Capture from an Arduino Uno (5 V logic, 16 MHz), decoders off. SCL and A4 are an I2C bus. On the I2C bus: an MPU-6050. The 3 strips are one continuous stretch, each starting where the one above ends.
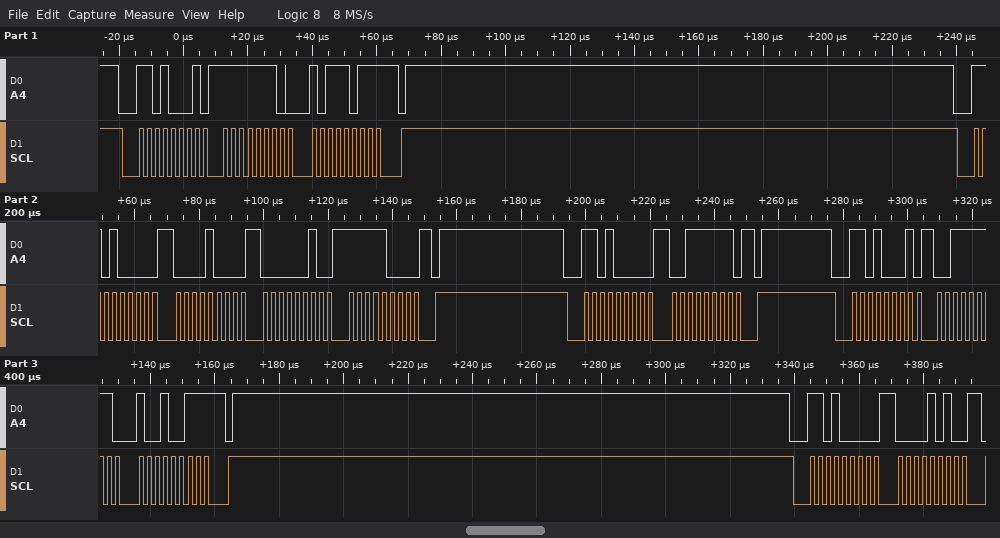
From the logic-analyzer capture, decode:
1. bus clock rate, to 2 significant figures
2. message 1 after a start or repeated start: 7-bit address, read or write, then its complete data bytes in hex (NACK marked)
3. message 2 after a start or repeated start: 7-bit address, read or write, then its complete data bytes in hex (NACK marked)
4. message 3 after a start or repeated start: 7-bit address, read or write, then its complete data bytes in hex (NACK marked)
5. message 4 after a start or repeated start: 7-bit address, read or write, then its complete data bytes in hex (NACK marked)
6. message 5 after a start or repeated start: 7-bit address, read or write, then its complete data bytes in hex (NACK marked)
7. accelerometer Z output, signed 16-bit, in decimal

400 kHz
0x68 read: FE BB NACK
0x68 write: 08 02 F8
0x68 write: 3F
0x68 read: 3F 93 NACK
0x68 write: 0A
16275
